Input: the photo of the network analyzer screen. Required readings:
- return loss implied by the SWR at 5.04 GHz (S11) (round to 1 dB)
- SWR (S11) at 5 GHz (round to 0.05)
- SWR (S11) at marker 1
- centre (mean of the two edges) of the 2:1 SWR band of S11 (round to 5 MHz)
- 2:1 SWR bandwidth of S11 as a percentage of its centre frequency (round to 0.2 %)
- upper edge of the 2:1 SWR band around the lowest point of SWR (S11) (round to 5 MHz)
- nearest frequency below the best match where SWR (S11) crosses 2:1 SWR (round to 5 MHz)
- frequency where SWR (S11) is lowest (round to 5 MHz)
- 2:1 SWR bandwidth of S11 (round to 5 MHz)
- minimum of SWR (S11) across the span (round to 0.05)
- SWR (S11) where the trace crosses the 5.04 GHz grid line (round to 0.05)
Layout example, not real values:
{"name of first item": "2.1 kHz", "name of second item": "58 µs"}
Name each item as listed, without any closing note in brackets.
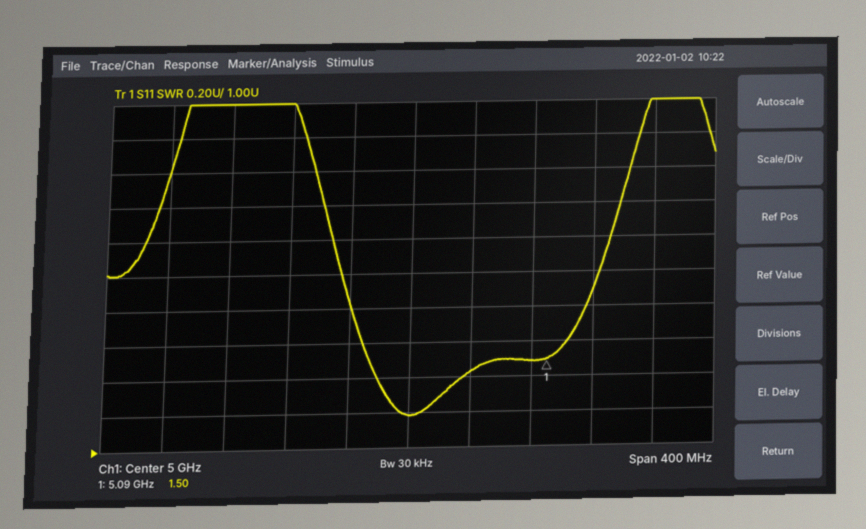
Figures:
{"return loss implied by the SWR at 5.04 GHz (S11)": "15 dB", "SWR (S11) at 5 GHz": "1.20", "SWR (S11) at marker 1": "1.50", "centre (mean of the two edges) of the 2:1 SWR band of S11": "5.040 GHz", "2:1 SWR bandwidth of S11 as a percentage of its centre frequency": "3.4 %", "upper edge of the 2:1 SWR band around the lowest point of SWR (S11)": "5.125 GHz", "nearest frequency below the best match where SWR (S11) crosses 2:1 SWR": "4.955 GHz", "frequency where SWR (S11) is lowest": "5.000 GHz", "2:1 SWR bandwidth of S11": "170 MHz", "minimum of SWR (S11) across the span": "1.20", "SWR (S11) where the trace crosses the 5.04 GHz grid line": "1.45"}
